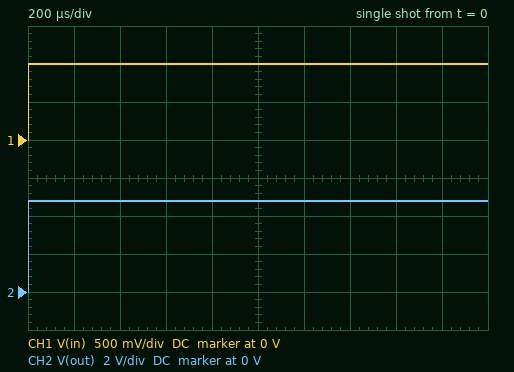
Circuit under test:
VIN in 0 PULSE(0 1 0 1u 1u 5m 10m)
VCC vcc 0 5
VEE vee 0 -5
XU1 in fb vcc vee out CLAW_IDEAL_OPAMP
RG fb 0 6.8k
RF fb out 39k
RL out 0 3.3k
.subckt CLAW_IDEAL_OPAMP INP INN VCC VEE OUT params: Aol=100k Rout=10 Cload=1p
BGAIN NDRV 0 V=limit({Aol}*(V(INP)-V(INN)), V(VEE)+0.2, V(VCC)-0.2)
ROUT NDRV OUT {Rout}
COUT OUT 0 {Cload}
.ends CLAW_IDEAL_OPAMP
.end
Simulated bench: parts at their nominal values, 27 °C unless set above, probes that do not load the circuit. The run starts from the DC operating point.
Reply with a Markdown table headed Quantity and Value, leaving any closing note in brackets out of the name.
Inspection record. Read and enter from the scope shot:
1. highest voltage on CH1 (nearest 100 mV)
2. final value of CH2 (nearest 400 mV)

| Quantity | Value |
|---|---|
| highest voltage on CH1 | 1.0 V |
| final value of CH2 | 4.8 V |
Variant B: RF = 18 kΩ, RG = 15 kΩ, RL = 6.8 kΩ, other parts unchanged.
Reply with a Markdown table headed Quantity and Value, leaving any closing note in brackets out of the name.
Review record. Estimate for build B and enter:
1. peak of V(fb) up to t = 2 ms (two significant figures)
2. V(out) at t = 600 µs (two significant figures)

| Quantity | Value |
|---|---|
| peak of V(fb) up to t = 2 ms | 1.0 V |
| V(out) at t = 600 µs | 2.2 V |
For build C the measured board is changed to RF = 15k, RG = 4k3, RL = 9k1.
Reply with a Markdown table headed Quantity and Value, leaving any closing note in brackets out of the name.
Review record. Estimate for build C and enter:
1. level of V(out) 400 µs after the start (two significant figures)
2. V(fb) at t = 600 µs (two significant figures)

| Quantity | Value |
|---|---|
| level of V(out) 400 µs after the start | 4.5 V |
| V(fb) at t = 600 µs | 1.0 V |
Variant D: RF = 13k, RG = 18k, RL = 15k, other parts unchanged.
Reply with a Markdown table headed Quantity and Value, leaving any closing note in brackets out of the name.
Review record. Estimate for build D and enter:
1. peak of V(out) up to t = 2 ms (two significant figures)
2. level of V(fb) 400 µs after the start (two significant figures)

| Quantity | Value |
|---|---|
| peak of V(out) up to t = 2 ms | 1.7 V |
| level of V(fb) 400 µs after the start | 1.0 V |
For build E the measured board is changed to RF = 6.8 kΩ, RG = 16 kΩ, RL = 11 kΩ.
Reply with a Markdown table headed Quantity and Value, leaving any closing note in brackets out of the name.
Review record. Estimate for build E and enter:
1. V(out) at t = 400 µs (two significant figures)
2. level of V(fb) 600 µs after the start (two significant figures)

| Quantity | Value |
|---|---|
| V(out) at t = 400 µs | 1.4 V |
| level of V(fb) 600 µs after the start | 1.0 V |
